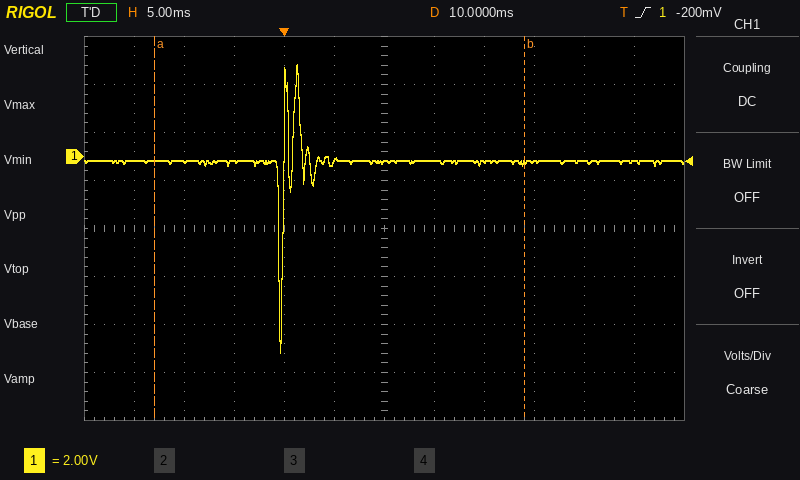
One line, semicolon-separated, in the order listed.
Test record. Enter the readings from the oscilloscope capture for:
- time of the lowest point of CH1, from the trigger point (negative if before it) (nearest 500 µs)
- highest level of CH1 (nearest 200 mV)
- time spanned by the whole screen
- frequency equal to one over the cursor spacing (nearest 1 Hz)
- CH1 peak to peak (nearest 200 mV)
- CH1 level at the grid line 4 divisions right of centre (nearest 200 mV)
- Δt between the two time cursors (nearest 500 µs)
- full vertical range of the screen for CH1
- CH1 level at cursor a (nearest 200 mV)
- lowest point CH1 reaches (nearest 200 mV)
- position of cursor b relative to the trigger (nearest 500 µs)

-500 µs; 3.8 V; 60 ms; 27 Hz; 12.0 V; -200 mV; 37.0 ms; 16 V; -200 mV; -8.2 V; +24.0 ms
